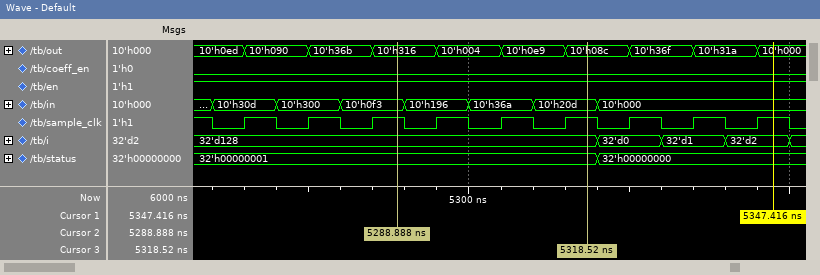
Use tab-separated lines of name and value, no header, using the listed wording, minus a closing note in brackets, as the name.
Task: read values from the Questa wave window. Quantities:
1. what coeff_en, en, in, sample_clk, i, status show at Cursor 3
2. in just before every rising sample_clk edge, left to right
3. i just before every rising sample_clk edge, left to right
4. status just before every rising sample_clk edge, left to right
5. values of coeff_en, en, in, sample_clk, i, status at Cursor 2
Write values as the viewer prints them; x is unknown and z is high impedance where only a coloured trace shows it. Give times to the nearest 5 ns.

what coeff_en, en, in, sample_clk, i, status show at Cursor 3	coeff_en=0, en=1, in=10'h20d, sample_clk=1, i=32'd128, status=32'h00000001
in just before every rising sample_clk edge, left to right	10'h30d, 10'h300, 10'h0f3, 10'h196, 10'h36a, 10'h20d, 10'h000, 10'h000, 10'h000
i just before every rising sample_clk edge, left to right	32'd128, 32'd128, 32'd128, 32'd128, 32'd128, 32'd128, 32'd0, 32'd1, 32'd2
status just before every rising sample_clk edge, left to right	32'h00000001, 32'h00000001, 32'h00000001, 32'h00000001, 32'h00000001, 32'h00000001, 32'h00000000, 32'h00000000, 32'h00000000
values of coeff_en, en, in, sample_clk, i, status at Cursor 2	coeff_en=0, en=1, in=10'h0f3, sample_clk=1, i=32'd128, status=32'h00000001
